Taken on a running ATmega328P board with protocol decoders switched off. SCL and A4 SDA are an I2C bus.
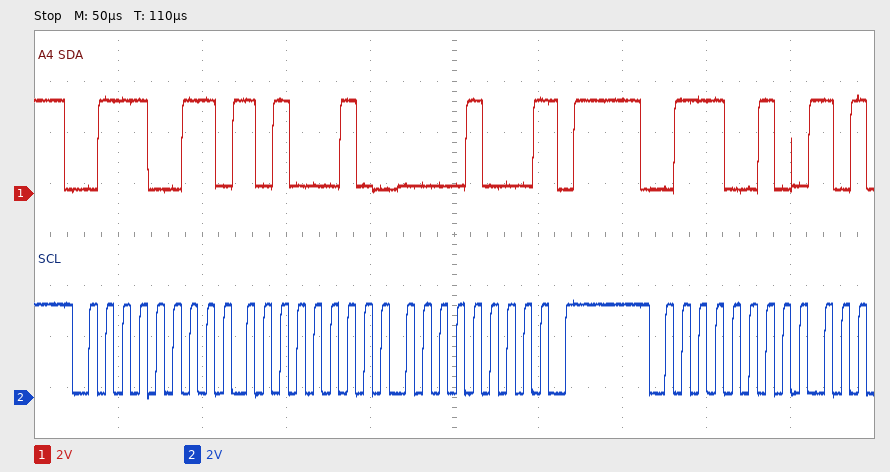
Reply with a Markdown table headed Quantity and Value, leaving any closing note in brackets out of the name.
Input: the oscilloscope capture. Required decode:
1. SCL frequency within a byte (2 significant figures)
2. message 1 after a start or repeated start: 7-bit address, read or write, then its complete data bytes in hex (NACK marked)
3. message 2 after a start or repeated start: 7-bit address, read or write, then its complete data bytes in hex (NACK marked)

| Quantity | Value |
|---|---|
| SCL frequency within a byte | 100 kHz |
| message 1 after a start or repeated start: 7-bit address, read or write, then its complete data bytes in hex | 0x39 read: A2 08 NACK |
| message 2 after a start or repeated start: 7-bit address, read or write, then its complete data bytes in hex | 0x39 write |
